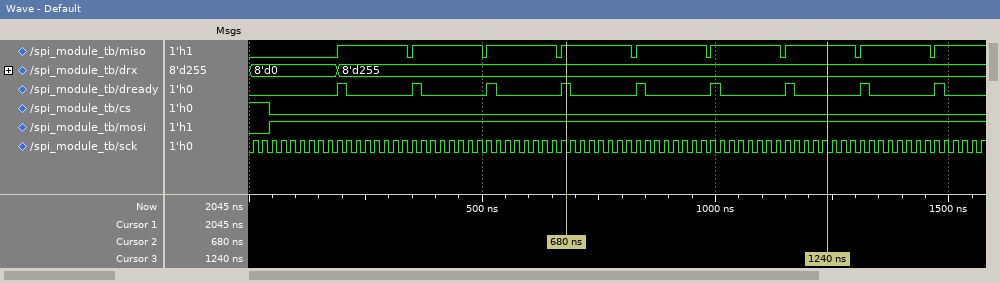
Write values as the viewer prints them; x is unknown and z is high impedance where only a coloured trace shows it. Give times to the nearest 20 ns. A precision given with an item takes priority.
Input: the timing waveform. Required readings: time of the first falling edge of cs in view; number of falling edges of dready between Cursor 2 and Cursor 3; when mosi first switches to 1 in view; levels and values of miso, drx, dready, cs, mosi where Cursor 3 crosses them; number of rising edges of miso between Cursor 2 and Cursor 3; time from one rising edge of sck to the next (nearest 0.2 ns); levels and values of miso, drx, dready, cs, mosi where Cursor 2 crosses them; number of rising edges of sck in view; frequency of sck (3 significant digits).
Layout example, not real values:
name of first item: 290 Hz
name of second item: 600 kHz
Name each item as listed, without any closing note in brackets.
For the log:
time of the first falling edge of cs in view: 40 ns
number of falling edges of dready between Cursor 2 and Cursor 3: 4
when mosi first switches to 1 in view: 40 ns
levels and values of miso, drx, dready, cs, mosi where Cursor 3 crosses them: miso=1, drx=8'd255, dready=0, cs=0, mosi=1
number of rising edges of miso between Cursor 2 and Cursor 3: 3
time from one rising edge of sck to the next: 20 ns
levels and values of miso, drx, dready, cs, mosi where Cursor 2 crosses them: miso=1, drx=8'd255, dready=1, cs=0, mosi=1
number of rising edges of sck in view: 79
frequency of sck: 50.0 MHz
